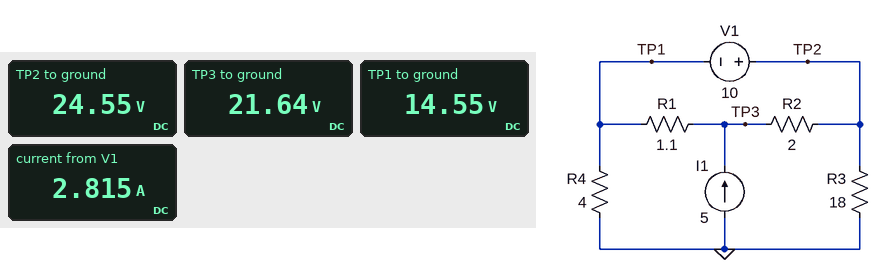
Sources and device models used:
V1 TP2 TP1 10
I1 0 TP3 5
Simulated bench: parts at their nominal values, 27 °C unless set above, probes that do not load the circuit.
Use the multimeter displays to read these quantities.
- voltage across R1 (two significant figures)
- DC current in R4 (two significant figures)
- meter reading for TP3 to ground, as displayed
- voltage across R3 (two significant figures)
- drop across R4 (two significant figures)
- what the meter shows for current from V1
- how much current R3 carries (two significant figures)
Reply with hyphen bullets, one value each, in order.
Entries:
- 7.1 V
- 3.6 A
- 21.64 V
- 25 V
- 15 V
- 2.815 A
- 1.4 A
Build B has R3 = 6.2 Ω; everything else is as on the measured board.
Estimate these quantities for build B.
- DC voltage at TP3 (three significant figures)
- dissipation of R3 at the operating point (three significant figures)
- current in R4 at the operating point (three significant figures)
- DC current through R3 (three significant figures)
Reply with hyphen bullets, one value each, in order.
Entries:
- 15.3 V
- 53.6 W
- 2.06 A
- 2.94 A
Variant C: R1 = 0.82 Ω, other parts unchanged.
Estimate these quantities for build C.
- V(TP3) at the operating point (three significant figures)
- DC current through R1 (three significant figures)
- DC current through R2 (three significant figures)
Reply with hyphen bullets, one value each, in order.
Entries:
- 20.4 V
- 7.09 A
- 2.09 A
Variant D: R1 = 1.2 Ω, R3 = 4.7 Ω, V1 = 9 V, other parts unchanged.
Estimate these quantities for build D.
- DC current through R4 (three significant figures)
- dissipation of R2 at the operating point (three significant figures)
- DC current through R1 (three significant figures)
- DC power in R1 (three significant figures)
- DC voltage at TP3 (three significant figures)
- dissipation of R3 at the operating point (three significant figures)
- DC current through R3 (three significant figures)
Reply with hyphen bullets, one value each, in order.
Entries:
- 1.67 A
- 1.76 W
- 5.94 A
- 42.3 W
- 13.8 V
- 52.2 W
- 3.33 A
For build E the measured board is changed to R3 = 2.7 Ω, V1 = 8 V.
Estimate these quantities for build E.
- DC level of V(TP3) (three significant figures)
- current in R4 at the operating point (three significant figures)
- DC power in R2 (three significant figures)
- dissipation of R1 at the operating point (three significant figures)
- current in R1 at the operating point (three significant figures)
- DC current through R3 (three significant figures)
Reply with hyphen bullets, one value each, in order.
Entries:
- 9.67 V
- 821 mA
- 1.30 W
- 37.1 W
- 5.81 A
- 4.18 A
